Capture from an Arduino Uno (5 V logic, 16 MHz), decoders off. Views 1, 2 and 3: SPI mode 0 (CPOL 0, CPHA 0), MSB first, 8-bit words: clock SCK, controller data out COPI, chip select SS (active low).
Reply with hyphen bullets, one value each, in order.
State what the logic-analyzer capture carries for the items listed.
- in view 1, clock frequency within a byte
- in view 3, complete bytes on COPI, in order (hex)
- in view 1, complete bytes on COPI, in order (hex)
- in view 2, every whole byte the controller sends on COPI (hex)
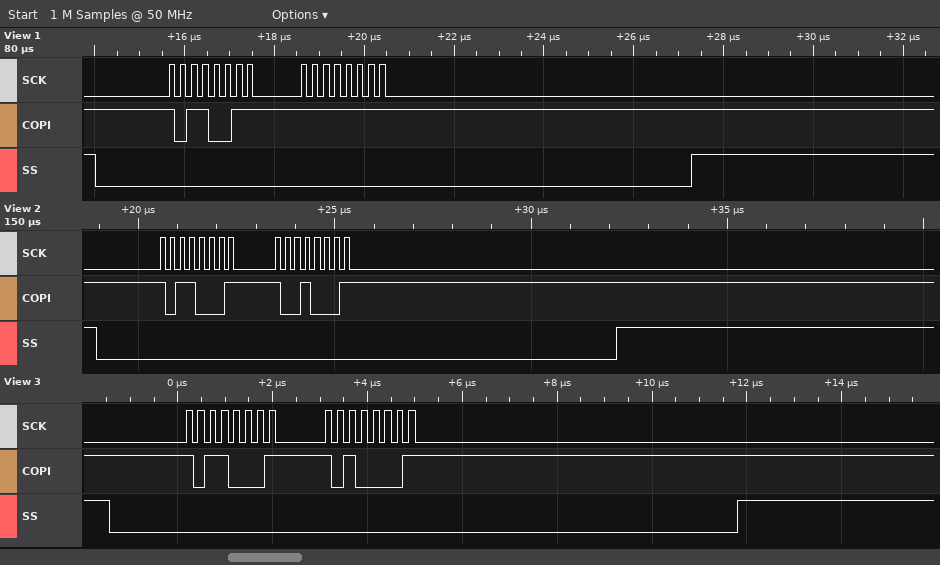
- 4 MHz
- B1 A1
- B3 FF
- B1 91
